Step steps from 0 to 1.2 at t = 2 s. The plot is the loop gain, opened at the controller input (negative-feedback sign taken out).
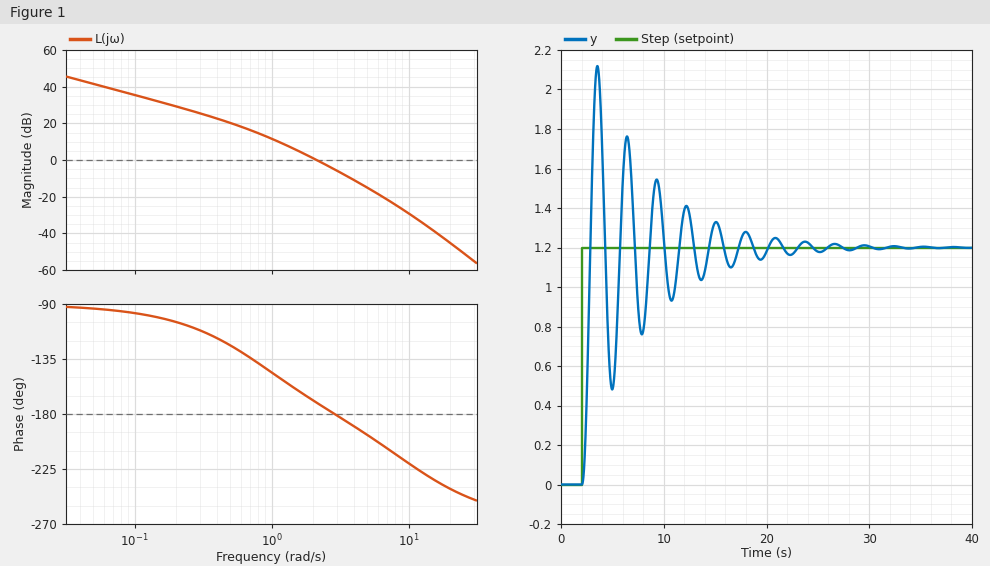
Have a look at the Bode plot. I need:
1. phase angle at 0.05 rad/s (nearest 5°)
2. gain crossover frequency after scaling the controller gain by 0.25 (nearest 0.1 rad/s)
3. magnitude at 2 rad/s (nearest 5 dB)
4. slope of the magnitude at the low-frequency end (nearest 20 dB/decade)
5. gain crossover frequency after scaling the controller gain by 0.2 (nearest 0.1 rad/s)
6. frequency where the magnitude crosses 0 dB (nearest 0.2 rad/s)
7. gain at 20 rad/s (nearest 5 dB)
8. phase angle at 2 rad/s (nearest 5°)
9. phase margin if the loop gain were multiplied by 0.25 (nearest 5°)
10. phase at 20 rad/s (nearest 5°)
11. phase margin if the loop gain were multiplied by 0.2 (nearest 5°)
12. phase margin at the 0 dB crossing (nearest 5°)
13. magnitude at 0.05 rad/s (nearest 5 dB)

-95°
1.0 rad/s
0 dB
-20 dB/decade
0.8 rad/s
2.2 rad/s
-45 dB
-170°
35°
-240°
40°
10°
40 dB
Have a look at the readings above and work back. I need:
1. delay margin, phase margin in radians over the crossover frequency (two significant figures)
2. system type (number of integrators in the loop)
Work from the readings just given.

0.079 s
1
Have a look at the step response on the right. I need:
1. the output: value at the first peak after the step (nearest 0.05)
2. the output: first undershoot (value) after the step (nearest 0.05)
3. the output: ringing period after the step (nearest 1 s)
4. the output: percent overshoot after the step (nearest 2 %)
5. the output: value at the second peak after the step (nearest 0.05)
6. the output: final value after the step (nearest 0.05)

2.10
0.50
3 s
76 %
1.75
1.20
